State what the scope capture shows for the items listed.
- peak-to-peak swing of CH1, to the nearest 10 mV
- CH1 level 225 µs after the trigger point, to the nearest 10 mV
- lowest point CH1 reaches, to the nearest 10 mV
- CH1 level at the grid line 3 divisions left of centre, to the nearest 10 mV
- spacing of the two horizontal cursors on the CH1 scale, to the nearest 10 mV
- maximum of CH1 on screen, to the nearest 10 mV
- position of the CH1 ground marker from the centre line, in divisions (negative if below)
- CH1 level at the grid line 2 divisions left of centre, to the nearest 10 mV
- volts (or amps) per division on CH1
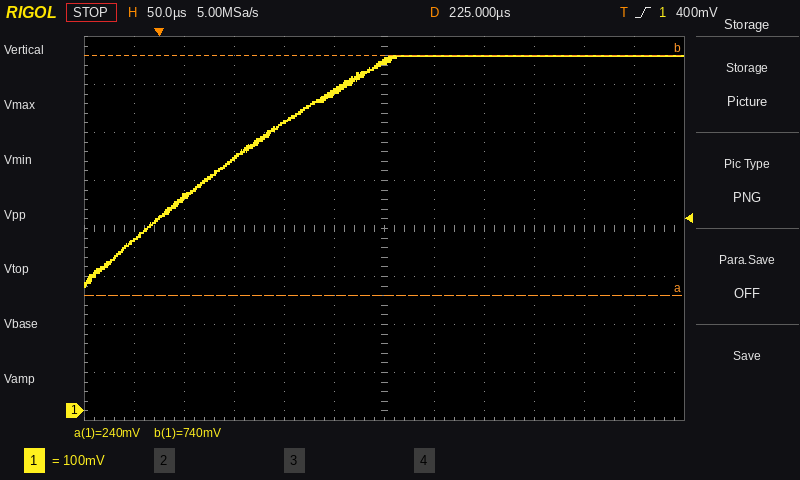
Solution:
480 mV
730 mV
260 mV
530 mV
500 mV
740 mV
-3.8 div
600 mV
100 mV
